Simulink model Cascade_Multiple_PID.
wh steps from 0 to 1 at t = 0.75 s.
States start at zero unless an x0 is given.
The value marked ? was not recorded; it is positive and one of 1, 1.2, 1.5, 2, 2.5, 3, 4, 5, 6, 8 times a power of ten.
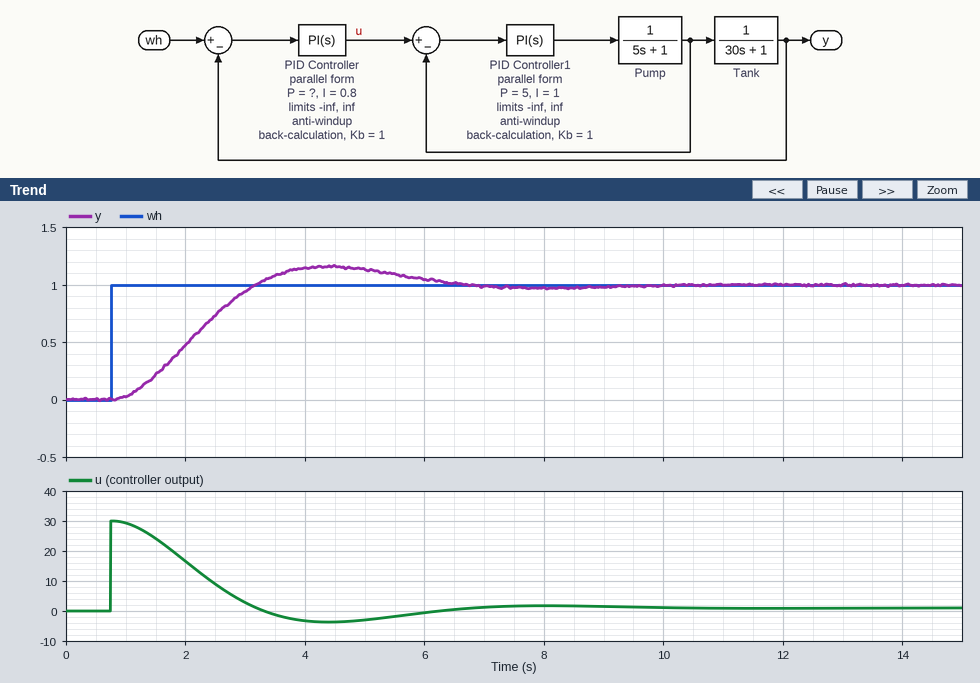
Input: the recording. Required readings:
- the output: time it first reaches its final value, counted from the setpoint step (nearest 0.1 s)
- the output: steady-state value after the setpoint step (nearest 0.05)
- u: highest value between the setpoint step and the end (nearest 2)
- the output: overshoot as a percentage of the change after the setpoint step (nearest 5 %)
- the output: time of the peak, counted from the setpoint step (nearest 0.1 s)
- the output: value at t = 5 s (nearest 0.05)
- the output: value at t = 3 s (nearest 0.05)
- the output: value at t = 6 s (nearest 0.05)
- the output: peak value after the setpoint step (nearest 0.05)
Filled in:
2.4 s
1.00
30
15 %
3.6 s
1.15
0.95
1.05
1.15
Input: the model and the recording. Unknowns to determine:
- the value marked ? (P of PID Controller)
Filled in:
30
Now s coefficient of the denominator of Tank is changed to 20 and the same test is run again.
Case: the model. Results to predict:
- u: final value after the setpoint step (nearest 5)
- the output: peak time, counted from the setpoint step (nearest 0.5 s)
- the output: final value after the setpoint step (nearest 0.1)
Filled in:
0
3.0 s
1.0
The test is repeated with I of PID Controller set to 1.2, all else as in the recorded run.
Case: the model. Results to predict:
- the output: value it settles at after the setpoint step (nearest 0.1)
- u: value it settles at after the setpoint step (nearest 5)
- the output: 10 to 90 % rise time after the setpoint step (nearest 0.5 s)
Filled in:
1.0
0
1.5 s
